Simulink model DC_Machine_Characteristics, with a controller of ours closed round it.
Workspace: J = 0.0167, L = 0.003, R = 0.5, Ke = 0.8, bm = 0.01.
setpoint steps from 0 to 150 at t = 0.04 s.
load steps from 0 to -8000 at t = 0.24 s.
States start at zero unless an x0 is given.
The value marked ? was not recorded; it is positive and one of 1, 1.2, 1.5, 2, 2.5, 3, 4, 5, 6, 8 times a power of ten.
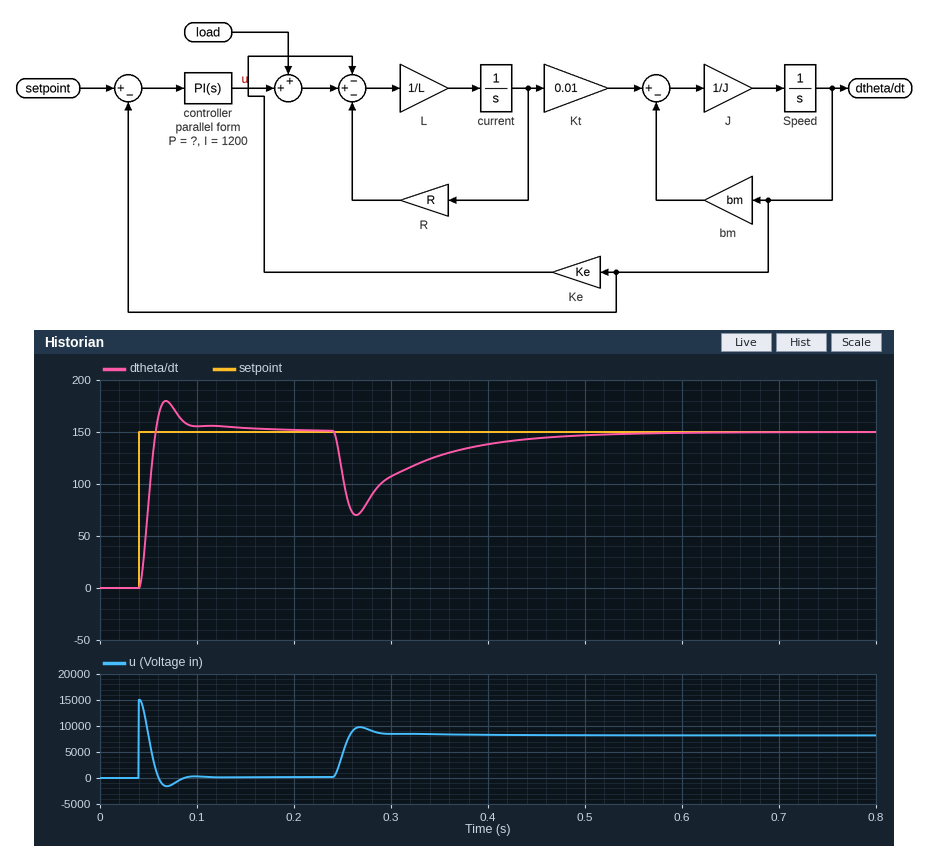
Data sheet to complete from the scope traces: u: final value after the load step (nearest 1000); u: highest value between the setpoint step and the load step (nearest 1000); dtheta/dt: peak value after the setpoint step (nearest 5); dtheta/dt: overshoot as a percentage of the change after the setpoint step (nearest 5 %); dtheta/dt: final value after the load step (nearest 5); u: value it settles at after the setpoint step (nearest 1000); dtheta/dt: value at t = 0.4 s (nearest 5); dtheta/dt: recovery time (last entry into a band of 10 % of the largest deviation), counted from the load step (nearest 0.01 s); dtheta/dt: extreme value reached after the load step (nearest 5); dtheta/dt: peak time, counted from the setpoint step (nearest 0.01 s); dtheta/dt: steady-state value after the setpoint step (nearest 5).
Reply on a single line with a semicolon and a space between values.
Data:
8000; 15000; 180; 20 %; 150; 0; 140; 0.19 s; 70; 0.03 s; 150
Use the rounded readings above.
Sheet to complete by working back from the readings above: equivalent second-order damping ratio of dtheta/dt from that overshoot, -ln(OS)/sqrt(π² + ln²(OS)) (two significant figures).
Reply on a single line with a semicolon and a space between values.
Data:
0.46
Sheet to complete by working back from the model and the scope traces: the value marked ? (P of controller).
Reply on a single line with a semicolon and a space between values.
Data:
100
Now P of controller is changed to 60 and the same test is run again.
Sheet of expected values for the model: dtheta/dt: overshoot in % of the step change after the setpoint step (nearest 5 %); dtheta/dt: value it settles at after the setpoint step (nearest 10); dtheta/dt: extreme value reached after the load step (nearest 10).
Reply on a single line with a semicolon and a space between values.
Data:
25 %; 150; 40
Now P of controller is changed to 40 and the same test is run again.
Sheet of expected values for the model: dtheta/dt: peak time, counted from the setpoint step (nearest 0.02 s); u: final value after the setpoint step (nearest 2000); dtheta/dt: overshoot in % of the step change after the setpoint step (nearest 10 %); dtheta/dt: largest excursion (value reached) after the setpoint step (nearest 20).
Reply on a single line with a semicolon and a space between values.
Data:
0.06 s; 0; 30 %; 200
